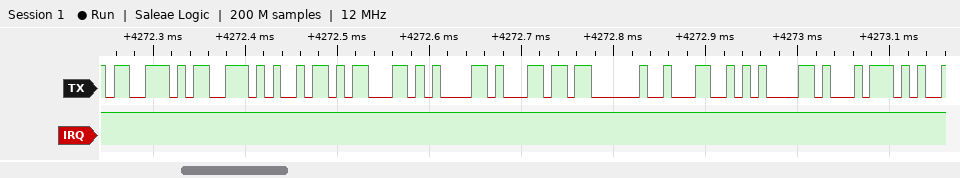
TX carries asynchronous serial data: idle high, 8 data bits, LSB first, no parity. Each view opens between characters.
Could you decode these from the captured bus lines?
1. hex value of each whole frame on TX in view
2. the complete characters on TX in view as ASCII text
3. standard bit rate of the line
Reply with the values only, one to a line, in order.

73, 73, 69, 63, 61, 6C, 20, 4C, 61, 74
"ssical Lat"
115200 baud
